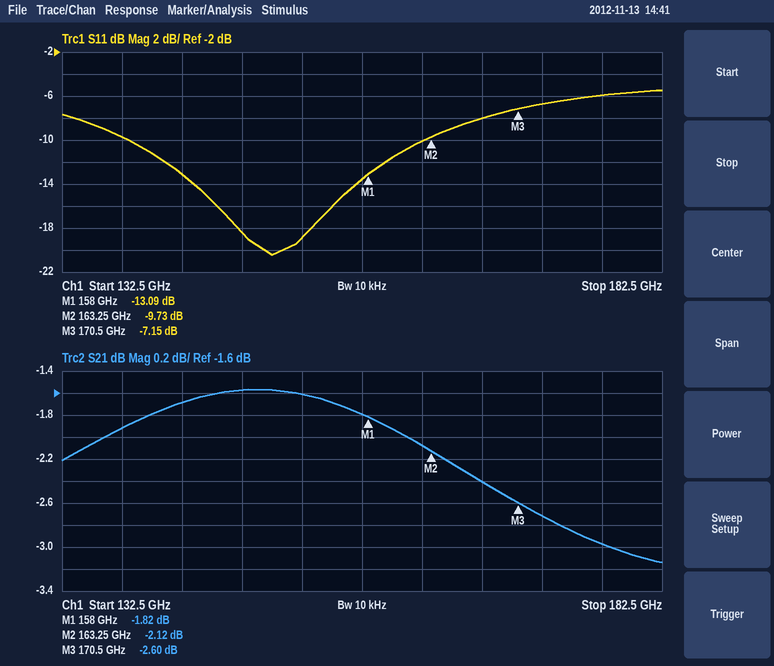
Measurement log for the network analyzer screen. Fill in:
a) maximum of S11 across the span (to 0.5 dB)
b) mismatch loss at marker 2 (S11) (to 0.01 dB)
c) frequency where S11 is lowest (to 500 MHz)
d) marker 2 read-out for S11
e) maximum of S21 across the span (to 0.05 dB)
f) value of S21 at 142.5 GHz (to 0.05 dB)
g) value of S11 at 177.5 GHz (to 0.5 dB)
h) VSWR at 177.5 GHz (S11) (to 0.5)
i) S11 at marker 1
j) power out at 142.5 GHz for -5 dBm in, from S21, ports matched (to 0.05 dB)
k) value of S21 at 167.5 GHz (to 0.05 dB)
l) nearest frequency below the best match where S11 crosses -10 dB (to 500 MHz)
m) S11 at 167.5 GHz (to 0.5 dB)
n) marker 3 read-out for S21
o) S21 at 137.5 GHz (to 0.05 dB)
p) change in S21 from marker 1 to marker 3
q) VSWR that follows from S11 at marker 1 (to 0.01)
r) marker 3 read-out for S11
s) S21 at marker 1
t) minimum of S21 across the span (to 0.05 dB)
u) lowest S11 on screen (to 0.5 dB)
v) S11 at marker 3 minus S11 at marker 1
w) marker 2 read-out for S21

-5.5 dB
0.49 dB
150.0 GHz
-9.73 dB
-1.55 dB
-1.70 dB
-6.0 dB
3.0
-13.09 dB
-6.70 dBm
-2.40 dB
138.0 GHz
-8.0 dB
-2.60 dB
-1.90 dB
-0.78 dB
1.57
-7.15 dB
-1.82 dB
-3.15 dB
-20.5 dB
5.94 dB
-2.12 dB
